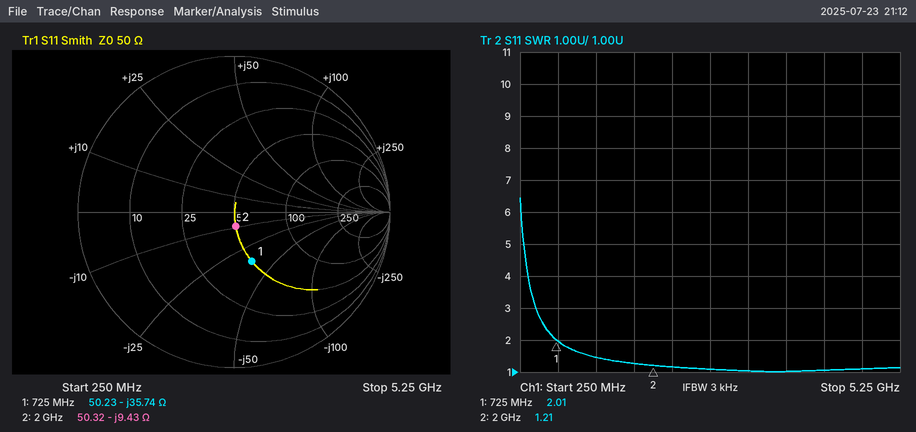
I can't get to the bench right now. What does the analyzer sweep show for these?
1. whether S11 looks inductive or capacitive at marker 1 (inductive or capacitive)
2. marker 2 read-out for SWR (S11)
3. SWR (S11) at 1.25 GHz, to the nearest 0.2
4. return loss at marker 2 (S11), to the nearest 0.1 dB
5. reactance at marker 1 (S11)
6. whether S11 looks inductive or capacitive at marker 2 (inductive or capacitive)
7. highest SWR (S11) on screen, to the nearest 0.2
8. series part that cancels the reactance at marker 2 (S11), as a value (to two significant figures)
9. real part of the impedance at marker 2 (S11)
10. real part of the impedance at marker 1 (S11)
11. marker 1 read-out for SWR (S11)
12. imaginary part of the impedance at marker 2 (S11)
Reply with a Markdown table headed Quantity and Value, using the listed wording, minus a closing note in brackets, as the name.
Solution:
| Quantity | Value |
|---|---|
| whether S11 looks inductive or capacitive at marker 1 | capacitive |
| marker 2 read-out for SWR | 1.21 |
| SWR (S11) at 1.25 GHz, to the nearest 0.2 | 1.4 |
| return loss at marker 2 (S11), to the nearest 0.1 dB | 20.6 dB |
| reactance at marker 1 | -35.74 Ω |
| whether S11 looks inductive or capacitive at marker 2 | capacitive |
| highest SWR (S11) on screen, to the nearest 0.2 | 6.4 |
| series part that cancels the reactance at marker 2 (S11), as a value | 750 pH |
| real part of the impedance at marker 2 | 50.32 Ω |
| real part of the impedance at marker 1 | 50.23 Ω |
| marker 1 read-out for SWR | 2.01 |
| imaginary part of the impedance at marker 2 | -9.43 Ω |
